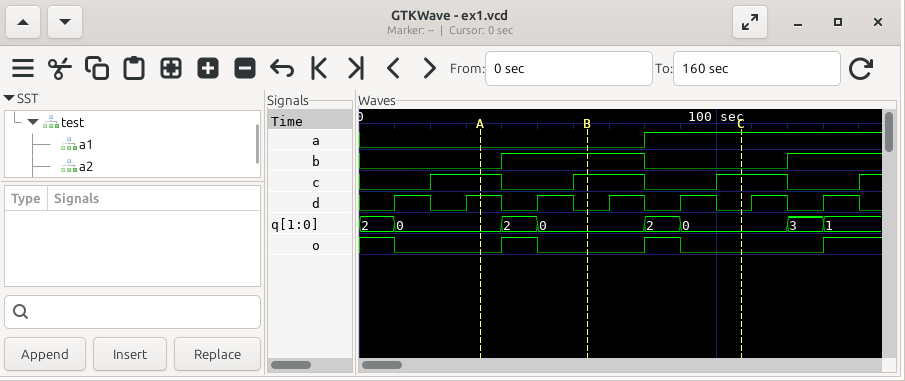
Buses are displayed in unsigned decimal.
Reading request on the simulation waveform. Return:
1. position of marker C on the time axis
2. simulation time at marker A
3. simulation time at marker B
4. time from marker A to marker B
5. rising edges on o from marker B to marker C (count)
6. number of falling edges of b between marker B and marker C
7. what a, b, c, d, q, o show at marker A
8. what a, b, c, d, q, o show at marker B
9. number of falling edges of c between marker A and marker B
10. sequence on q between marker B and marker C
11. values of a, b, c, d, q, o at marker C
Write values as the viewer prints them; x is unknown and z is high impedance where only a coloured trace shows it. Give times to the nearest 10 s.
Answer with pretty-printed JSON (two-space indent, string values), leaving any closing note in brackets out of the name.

{
  "position of marker C on the time axis": "110 s",
  "simulation time at marker A": "30 s",
  "simulation time at marker B": "60 s",
  "time from marker A to marker B": "30 s",
  "rising edges on o from marker B to marker C": "1",
  "number of falling edges of b between marker B and marker C": "1",
  "what a, b, c, d, q, o show at marker A": "a=0, b=0, c=1, d=1, q=0, o=0",
  "what a, b, c, d, q, o show at marker B": "a=0, b=1, c=1, d=0, q=0, o=0",
  "number of falling edges of c between marker A and marker B": "1",
  "sequence on q between marker B and marker C": "0, 2, 0",
  "values of a, b, c, d, q, o at marker C": "a=1, b=0, c=1, d=0, q=0, o=0"
}
